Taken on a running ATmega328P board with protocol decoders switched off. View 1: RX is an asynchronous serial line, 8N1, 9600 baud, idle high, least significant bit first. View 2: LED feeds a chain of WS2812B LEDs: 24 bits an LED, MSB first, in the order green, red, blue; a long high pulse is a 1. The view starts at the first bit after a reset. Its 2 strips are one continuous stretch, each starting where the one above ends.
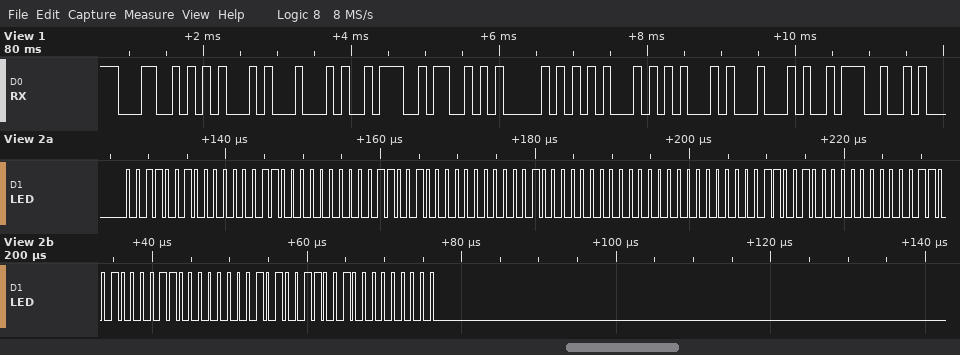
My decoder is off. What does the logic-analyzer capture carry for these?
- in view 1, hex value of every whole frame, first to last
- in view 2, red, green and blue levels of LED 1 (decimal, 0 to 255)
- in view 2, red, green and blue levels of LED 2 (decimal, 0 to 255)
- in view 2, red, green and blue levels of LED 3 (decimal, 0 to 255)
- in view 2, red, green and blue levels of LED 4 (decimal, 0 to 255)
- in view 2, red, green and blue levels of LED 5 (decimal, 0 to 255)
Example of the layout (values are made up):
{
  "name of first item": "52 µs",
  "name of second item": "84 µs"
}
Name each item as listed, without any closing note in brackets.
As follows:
{
  "in view 1, hex value of every whole frame, first to last": "4C 45 44 3A 53 50 45 45 44 3A",
  "in view 2, red, green and blue levels of LED 1": "3, 50, 0",
  "in view 2, red, green and blue levels of LED 2": "0, 50, 32",
  "in view 2, red, green and blue levels of LED 3": "0, 0, 50",
  "in view 2, red, green and blue levels of LED 4": "50, 0, 24",
  "in view 2, red, green and blue levels of LED 5": "50, 5, 0"
}
